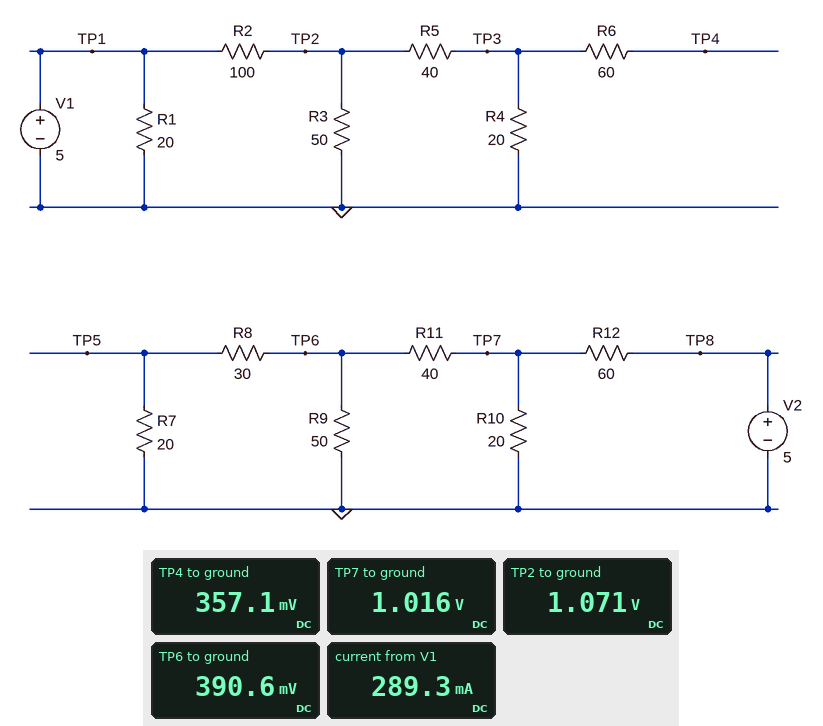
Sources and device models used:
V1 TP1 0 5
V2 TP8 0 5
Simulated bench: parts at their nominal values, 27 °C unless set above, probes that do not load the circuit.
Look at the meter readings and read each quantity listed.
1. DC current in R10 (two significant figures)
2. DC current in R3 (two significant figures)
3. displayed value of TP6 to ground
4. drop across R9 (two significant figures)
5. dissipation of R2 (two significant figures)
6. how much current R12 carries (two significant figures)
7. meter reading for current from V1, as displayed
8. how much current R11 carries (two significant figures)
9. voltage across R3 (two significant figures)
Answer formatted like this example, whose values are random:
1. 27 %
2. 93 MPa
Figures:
1. 51 mA
2. 21 mA
3. 390.6 mV
4. 390 mV
5. 150 mW
6. 66 mA
7. 289.3 mA
8. 16 mA
9. 1.1 V
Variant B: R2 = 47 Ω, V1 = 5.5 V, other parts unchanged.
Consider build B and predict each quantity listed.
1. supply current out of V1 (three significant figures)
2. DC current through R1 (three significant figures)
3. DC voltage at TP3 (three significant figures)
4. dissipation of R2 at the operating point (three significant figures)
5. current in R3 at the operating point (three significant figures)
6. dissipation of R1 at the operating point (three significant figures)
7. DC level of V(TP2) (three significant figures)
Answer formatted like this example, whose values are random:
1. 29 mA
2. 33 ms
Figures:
1. 349 mA
2. 275 mA
3. 673 mV
4. 258 mW
5. 40.4 mA
6. 1.51 W
7. 2.02 V
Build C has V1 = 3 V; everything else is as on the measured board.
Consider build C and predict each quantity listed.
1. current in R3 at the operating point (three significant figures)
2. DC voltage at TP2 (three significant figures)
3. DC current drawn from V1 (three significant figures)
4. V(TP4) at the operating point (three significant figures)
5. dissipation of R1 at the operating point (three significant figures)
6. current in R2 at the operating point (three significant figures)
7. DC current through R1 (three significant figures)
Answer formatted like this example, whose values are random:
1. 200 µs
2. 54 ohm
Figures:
1. 12.9 mA
2. 643 mV
3. 174 mA
4. 214 mV
5. 450 mW
6. 23.6 mA
7. 150 mA
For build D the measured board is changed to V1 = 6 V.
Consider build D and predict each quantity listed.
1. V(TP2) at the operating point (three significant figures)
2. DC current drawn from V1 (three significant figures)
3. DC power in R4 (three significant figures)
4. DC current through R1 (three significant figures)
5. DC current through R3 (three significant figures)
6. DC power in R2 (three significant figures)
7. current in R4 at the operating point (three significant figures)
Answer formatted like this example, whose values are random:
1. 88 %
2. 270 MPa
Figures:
1. 1.29 V
2. 347 mA
3. 9.18 mW
4. 300 mA
5. 25.7 mA
6. 222 mW
7. 21.4 mA
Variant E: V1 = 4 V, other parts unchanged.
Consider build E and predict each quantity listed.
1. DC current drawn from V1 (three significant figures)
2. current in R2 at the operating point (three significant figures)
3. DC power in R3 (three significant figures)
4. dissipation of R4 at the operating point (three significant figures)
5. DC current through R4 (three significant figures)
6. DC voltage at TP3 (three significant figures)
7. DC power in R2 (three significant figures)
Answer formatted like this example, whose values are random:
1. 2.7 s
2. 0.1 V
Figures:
1. 231 mA
2. 31.4 mA
3. 14.7 mW
4. 4.08 mW
5. 14.3 mA
6. 286 mV
7. 98.8 mW
